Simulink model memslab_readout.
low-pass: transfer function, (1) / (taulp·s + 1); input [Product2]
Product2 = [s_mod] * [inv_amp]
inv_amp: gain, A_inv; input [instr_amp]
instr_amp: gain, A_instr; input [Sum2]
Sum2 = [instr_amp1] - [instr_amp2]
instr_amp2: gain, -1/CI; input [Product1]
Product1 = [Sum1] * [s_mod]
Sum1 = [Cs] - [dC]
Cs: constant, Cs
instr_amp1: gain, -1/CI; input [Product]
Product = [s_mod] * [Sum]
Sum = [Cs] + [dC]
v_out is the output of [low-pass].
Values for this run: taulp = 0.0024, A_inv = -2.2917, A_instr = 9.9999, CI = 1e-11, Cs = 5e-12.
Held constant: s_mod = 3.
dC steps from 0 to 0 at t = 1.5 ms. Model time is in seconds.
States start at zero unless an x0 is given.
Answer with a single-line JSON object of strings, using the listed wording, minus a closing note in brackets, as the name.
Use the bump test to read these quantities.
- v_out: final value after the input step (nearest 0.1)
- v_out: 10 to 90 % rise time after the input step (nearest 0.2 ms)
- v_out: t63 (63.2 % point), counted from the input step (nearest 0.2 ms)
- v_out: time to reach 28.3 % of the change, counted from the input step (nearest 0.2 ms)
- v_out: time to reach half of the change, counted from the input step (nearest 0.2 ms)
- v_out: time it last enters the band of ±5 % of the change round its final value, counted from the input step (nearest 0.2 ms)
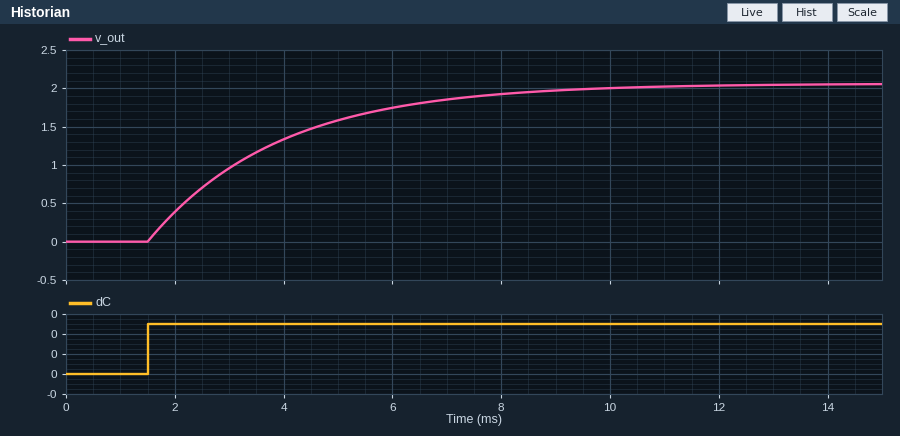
{"v_out: final value after the input step": "2.1", "v_out: 10 to 90 % rise time after the input step": "5.2 ms", "v_out: t63 (63.2 % point), counted from the input step": "2.4 ms", "v_out: time to reach 28.3 % of the change, counted from the input step": "0.8 ms", "v_out: time to reach half of the change, counted from the input step": "1.6 ms", "v_out: time it last enters the band of ±5 % of the change round its final value, counted from the input step": "7.2 ms"}
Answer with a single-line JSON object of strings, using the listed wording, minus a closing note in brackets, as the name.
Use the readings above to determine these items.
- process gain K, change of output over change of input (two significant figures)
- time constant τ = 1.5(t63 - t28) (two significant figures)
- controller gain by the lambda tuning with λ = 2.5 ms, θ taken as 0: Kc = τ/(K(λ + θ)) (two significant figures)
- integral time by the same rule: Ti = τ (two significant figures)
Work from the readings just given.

{"process gain K, change of output over change of input": "42000000000000", "time constant τ = 1.5(t63 - t28)": "2.4 ms", "controller gain by the lambda tuning with λ = 2.5 ms, θ taken as 0: Kc = τ/(K(λ + θ))": "0.000000000000023", "integral time by the same rule: Ti = τ": "2.4 ms"}
